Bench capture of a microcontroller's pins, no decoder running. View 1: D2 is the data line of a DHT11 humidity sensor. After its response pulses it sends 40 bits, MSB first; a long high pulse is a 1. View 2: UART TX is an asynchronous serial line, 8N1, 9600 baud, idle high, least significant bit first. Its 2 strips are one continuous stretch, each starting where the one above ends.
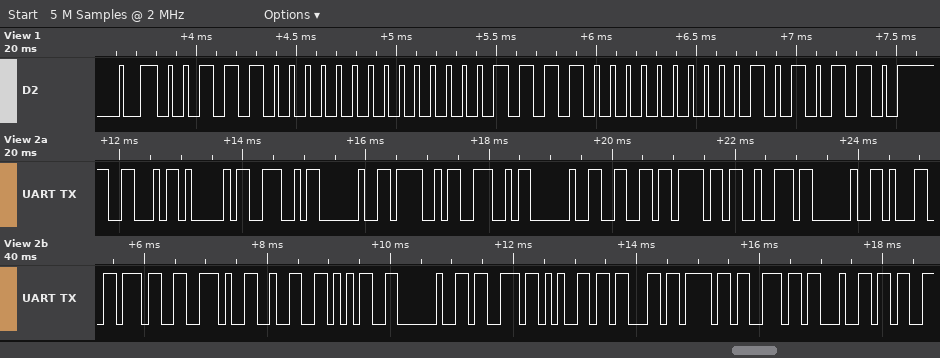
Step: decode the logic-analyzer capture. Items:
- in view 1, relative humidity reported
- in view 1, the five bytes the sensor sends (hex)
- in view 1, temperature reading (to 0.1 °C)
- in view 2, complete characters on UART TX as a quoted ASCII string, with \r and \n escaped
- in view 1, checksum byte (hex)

56 %
38 00 1E 00 56
30.0 °C
"FAN ON for 17.25 second"
0x56
